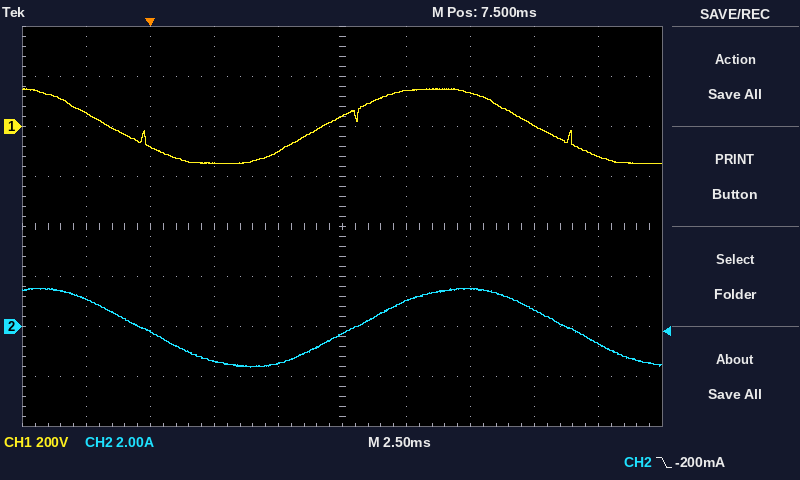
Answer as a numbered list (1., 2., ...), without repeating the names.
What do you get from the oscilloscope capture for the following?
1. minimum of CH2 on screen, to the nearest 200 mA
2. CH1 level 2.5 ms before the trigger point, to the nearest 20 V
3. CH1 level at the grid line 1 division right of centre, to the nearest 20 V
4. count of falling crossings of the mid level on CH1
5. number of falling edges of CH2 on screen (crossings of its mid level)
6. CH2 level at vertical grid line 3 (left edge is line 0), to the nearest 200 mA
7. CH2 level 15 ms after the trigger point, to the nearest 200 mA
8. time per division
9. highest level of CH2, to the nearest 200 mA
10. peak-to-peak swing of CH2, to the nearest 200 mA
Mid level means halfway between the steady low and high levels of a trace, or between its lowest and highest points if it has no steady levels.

1. -1.6 A
2. 60 V
3. 140 V
4. 2
5. 2
6. -1.4 A
7. 600 mA
8. 2.5 ms
9. 1.6 A
10. 3.2 A
